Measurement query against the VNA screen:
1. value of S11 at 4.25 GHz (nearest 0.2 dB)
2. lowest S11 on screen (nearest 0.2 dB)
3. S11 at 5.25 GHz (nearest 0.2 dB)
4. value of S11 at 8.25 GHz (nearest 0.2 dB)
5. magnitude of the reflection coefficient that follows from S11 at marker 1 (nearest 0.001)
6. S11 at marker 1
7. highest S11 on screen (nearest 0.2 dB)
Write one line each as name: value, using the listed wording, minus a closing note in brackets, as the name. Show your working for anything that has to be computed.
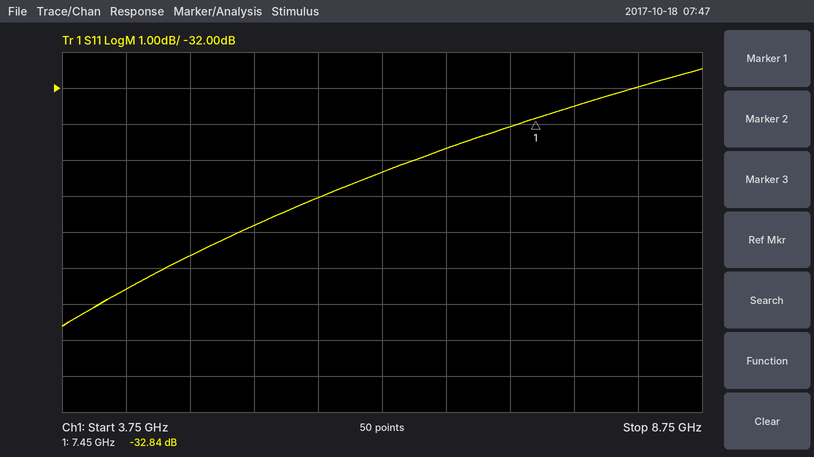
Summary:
value of S11 at 4.25 GHz: -37.6 dB
lowest S11 on screen: -38.6 dB
S11 at 5.25 GHz: -35.8 dB
value of S11 at 8.25 GHz: -32.0 dB
magnitude of the reflection coefficient that follows from S11 at marker 1: 10^(-32.84/20) ≈ 0.023
S11 at marker 1: -32.84 dB
highest S11 on screen: -31.4 dB
